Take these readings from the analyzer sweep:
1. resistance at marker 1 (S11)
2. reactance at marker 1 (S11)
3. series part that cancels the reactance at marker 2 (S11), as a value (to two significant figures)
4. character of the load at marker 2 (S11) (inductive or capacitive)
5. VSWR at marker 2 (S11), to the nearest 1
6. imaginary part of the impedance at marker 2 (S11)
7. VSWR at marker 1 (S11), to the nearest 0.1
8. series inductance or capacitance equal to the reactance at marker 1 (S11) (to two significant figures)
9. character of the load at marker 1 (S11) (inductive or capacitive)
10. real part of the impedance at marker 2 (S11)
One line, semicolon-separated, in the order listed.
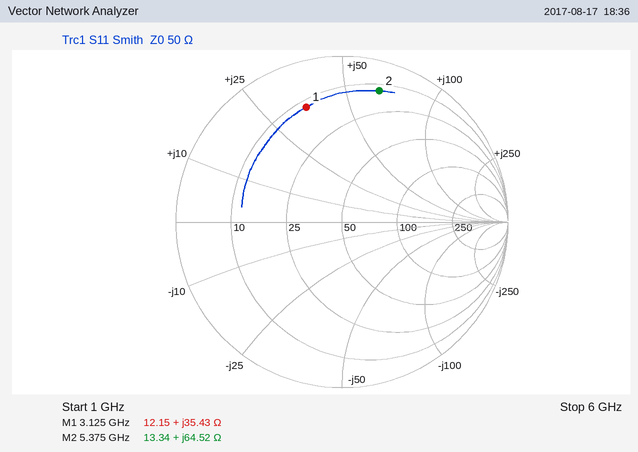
12.15 Ω; +35.43 Ω; 460 fF; inductive; 10; +64.52 Ω; 6.3; 1.8 nH; inductive; 13.34 Ω
